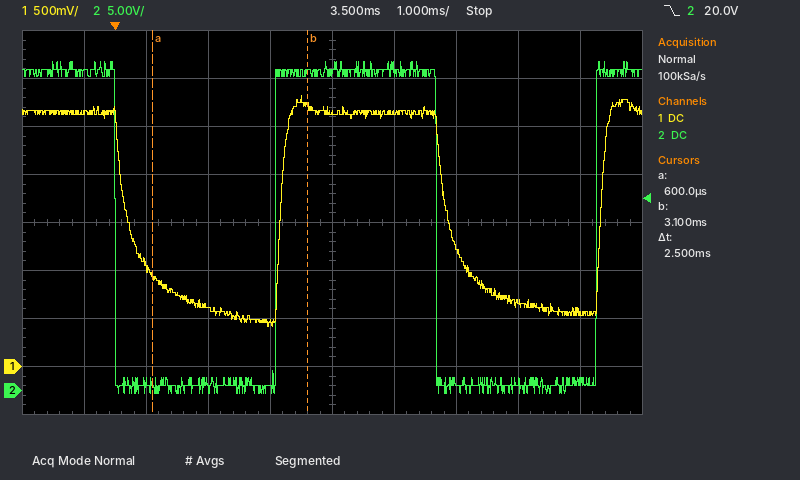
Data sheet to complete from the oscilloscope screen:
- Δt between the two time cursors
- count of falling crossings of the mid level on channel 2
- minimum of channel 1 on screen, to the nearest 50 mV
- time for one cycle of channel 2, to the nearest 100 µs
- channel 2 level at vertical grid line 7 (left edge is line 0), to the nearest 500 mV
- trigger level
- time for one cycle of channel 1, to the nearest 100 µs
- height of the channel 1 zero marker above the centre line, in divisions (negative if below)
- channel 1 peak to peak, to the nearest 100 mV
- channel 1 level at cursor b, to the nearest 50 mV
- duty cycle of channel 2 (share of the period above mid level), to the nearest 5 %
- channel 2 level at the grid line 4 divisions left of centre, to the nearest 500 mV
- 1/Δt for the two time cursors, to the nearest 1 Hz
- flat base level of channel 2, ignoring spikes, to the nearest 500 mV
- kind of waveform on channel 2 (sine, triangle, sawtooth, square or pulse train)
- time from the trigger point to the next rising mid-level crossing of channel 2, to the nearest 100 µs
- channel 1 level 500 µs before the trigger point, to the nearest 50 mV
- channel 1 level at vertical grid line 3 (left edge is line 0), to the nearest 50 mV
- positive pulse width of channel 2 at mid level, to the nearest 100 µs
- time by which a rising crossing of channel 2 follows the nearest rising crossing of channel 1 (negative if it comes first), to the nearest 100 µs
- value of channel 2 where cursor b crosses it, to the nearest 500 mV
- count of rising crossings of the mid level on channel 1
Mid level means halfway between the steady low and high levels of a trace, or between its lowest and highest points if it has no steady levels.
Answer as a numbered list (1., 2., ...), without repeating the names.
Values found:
1. 2.5 ms
2. 2
3. 400 mV
4. 5.2 ms
5. 1.0 V
6. 20.0 V
7. 5.2 ms
8. -3.0 div
9. 2.40 V
10. 2.70 V
11. 50 %
12. 33.0 V
13. 400 Hz
14. 500 mV
15. square
16. 2.6 ms
17. 2.65 V
18. 600 mV
19. 2.6 ms
20. -100 µs
21. 33.0 V
22. 2
